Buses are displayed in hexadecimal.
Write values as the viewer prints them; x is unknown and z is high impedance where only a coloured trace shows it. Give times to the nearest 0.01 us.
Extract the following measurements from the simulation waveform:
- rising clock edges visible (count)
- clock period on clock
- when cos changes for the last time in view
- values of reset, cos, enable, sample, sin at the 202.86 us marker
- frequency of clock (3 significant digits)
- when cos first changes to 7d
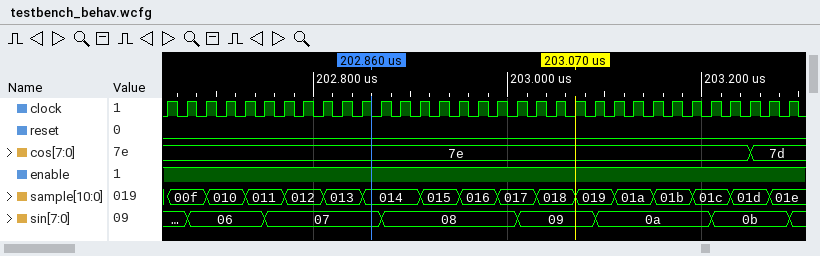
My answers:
33
0.02 us
203.25 us
reset=0, cos=7e, enable=1, sample=014, sin=07
50.0 MHz
203.25 us
